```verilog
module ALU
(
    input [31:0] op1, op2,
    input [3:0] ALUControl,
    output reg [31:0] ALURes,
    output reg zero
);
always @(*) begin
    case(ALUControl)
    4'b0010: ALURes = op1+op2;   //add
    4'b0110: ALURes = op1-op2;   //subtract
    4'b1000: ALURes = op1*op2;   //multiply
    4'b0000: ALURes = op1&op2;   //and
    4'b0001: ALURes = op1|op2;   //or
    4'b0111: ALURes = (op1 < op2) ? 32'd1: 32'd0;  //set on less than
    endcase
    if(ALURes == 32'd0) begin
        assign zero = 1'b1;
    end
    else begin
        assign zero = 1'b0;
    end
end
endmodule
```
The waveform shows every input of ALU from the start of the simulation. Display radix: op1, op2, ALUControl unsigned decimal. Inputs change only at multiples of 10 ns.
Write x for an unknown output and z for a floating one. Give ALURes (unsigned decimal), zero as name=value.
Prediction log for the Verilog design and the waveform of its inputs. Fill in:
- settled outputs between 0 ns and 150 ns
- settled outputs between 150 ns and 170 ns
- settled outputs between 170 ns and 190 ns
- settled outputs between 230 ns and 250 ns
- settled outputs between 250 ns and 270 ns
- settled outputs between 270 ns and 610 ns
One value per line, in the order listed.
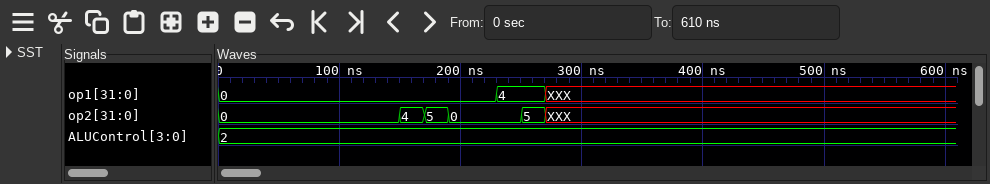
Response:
ALURes=0, zero=1
ALURes=4, zero=0
ALURes=5, zero=0
ALURes=4, zero=0
ALURes=9, zero=0
ALURes=x, zero=0
